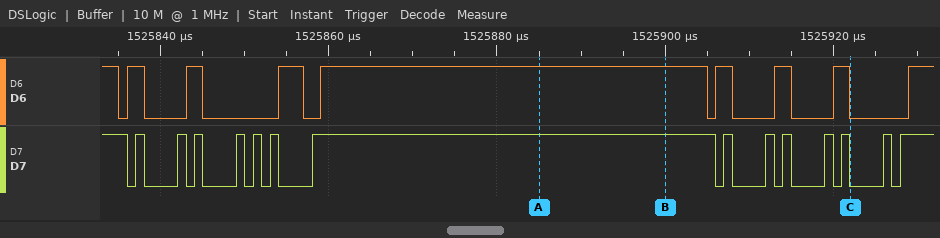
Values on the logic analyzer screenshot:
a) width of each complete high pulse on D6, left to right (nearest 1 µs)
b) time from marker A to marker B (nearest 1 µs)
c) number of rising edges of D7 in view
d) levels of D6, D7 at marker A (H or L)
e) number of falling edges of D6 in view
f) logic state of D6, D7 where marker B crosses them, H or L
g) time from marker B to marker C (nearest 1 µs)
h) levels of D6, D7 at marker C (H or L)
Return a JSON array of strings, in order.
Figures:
["2 µs, 2 µs, 3 µs, 46 µs, 2 µs, 2 µs, 2 µs", "15 µs", "14", "D6=H, D7=H", "8", "D6=H, D7=H", "22 µs", "D6=L, D7=L"]
